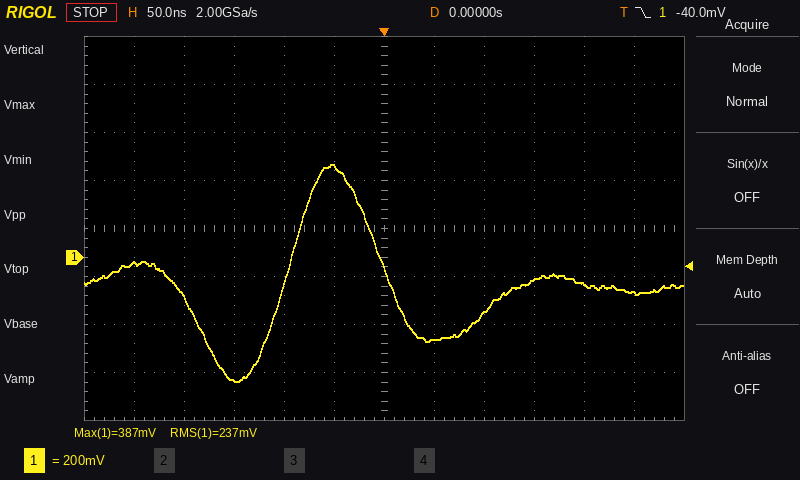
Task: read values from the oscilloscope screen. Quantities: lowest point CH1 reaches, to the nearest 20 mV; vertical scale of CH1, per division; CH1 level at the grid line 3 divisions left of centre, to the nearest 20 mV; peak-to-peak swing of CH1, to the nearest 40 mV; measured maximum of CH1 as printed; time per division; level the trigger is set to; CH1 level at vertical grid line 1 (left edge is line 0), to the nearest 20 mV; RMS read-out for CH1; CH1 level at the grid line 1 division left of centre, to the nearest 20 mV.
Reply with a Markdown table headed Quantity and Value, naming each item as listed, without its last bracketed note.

| Quantity | Value |
|---|---|
| lowest point CH1 reaches, to the nearest 20 mV | -520 mV |
| vertical scale of CH1, per division | 200 mV |
| CH1 level at the grid line 3 divisions left of centre, to the nearest 20 mV | -520 mV |
| peak-to-peak swing of CH1, to the nearest 40 mV | 920 mV |
| measured maximum of CH1 as printed | 387 mV |
| time per division | 50 ns |
| level the trigger is set to | -40.0 mV |
| CH1 level at vertical grid line 1 (left edge is line 0), to the nearest 20 mV | -20 mV |
| RMS read-out for CH1 | 237 mV |
| CH1 level at the grid line 1 division left of centre, to the nearest 20 mV | 380 mV |
